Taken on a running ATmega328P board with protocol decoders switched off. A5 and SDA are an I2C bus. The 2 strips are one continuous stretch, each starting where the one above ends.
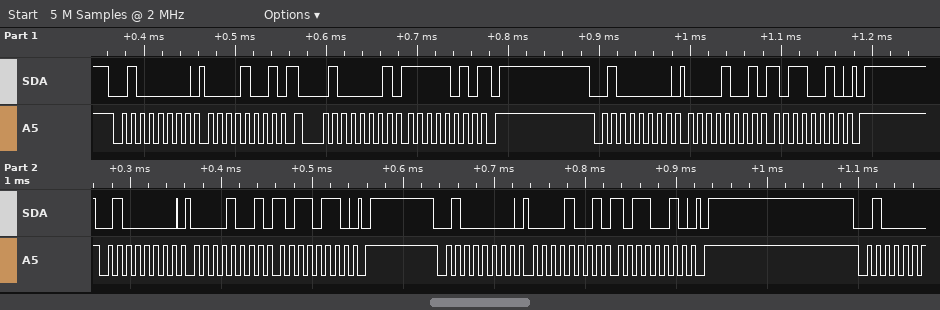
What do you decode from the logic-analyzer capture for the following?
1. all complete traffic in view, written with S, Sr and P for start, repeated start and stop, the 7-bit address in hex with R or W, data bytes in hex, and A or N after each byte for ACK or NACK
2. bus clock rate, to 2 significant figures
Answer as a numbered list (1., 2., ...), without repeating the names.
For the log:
1. S 20W A 09 A Sr 20R A FA N P S 20W A 09 A B2 A P S 20W A 09 A B6 A P S 20W A 09 A B2 A P
2. 100 kHz
